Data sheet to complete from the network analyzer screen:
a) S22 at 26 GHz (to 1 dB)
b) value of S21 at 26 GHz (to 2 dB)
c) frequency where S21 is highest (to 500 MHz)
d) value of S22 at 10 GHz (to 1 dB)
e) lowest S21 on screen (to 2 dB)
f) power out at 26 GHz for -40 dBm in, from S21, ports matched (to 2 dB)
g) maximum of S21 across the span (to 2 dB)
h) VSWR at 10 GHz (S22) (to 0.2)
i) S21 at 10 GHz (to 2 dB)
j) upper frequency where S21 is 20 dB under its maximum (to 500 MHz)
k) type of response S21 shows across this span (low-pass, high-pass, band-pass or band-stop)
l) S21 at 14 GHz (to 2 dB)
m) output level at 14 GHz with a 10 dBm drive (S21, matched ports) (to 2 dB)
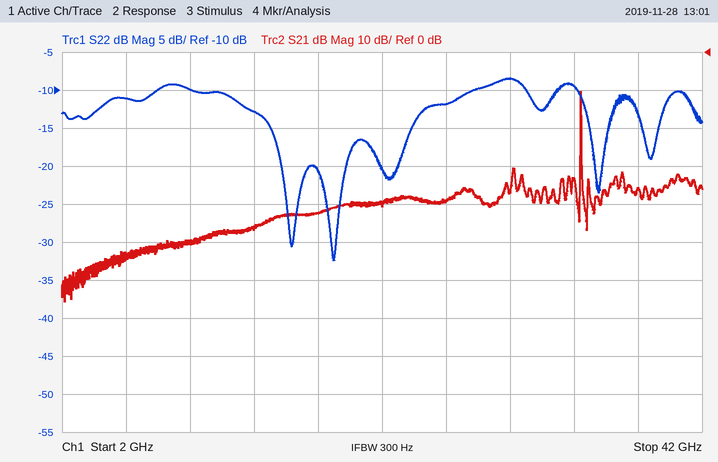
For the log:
-12 dB
-40 dB
34.5 GHz
-10 dB
-66 dB
-80 dBm
-10 dB
2.0
-50 dB
34.5 GHz
band-pass
-46 dB
-36 dBm
